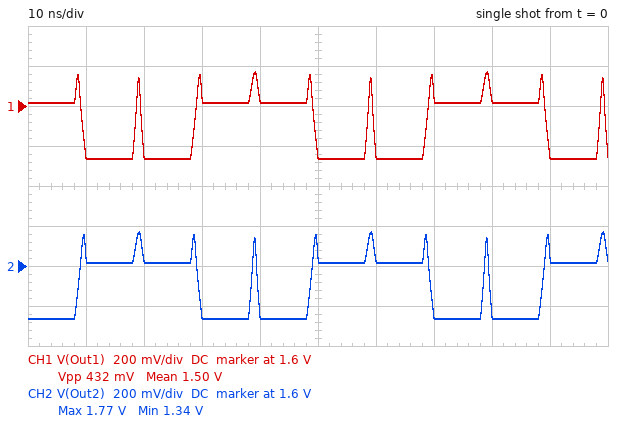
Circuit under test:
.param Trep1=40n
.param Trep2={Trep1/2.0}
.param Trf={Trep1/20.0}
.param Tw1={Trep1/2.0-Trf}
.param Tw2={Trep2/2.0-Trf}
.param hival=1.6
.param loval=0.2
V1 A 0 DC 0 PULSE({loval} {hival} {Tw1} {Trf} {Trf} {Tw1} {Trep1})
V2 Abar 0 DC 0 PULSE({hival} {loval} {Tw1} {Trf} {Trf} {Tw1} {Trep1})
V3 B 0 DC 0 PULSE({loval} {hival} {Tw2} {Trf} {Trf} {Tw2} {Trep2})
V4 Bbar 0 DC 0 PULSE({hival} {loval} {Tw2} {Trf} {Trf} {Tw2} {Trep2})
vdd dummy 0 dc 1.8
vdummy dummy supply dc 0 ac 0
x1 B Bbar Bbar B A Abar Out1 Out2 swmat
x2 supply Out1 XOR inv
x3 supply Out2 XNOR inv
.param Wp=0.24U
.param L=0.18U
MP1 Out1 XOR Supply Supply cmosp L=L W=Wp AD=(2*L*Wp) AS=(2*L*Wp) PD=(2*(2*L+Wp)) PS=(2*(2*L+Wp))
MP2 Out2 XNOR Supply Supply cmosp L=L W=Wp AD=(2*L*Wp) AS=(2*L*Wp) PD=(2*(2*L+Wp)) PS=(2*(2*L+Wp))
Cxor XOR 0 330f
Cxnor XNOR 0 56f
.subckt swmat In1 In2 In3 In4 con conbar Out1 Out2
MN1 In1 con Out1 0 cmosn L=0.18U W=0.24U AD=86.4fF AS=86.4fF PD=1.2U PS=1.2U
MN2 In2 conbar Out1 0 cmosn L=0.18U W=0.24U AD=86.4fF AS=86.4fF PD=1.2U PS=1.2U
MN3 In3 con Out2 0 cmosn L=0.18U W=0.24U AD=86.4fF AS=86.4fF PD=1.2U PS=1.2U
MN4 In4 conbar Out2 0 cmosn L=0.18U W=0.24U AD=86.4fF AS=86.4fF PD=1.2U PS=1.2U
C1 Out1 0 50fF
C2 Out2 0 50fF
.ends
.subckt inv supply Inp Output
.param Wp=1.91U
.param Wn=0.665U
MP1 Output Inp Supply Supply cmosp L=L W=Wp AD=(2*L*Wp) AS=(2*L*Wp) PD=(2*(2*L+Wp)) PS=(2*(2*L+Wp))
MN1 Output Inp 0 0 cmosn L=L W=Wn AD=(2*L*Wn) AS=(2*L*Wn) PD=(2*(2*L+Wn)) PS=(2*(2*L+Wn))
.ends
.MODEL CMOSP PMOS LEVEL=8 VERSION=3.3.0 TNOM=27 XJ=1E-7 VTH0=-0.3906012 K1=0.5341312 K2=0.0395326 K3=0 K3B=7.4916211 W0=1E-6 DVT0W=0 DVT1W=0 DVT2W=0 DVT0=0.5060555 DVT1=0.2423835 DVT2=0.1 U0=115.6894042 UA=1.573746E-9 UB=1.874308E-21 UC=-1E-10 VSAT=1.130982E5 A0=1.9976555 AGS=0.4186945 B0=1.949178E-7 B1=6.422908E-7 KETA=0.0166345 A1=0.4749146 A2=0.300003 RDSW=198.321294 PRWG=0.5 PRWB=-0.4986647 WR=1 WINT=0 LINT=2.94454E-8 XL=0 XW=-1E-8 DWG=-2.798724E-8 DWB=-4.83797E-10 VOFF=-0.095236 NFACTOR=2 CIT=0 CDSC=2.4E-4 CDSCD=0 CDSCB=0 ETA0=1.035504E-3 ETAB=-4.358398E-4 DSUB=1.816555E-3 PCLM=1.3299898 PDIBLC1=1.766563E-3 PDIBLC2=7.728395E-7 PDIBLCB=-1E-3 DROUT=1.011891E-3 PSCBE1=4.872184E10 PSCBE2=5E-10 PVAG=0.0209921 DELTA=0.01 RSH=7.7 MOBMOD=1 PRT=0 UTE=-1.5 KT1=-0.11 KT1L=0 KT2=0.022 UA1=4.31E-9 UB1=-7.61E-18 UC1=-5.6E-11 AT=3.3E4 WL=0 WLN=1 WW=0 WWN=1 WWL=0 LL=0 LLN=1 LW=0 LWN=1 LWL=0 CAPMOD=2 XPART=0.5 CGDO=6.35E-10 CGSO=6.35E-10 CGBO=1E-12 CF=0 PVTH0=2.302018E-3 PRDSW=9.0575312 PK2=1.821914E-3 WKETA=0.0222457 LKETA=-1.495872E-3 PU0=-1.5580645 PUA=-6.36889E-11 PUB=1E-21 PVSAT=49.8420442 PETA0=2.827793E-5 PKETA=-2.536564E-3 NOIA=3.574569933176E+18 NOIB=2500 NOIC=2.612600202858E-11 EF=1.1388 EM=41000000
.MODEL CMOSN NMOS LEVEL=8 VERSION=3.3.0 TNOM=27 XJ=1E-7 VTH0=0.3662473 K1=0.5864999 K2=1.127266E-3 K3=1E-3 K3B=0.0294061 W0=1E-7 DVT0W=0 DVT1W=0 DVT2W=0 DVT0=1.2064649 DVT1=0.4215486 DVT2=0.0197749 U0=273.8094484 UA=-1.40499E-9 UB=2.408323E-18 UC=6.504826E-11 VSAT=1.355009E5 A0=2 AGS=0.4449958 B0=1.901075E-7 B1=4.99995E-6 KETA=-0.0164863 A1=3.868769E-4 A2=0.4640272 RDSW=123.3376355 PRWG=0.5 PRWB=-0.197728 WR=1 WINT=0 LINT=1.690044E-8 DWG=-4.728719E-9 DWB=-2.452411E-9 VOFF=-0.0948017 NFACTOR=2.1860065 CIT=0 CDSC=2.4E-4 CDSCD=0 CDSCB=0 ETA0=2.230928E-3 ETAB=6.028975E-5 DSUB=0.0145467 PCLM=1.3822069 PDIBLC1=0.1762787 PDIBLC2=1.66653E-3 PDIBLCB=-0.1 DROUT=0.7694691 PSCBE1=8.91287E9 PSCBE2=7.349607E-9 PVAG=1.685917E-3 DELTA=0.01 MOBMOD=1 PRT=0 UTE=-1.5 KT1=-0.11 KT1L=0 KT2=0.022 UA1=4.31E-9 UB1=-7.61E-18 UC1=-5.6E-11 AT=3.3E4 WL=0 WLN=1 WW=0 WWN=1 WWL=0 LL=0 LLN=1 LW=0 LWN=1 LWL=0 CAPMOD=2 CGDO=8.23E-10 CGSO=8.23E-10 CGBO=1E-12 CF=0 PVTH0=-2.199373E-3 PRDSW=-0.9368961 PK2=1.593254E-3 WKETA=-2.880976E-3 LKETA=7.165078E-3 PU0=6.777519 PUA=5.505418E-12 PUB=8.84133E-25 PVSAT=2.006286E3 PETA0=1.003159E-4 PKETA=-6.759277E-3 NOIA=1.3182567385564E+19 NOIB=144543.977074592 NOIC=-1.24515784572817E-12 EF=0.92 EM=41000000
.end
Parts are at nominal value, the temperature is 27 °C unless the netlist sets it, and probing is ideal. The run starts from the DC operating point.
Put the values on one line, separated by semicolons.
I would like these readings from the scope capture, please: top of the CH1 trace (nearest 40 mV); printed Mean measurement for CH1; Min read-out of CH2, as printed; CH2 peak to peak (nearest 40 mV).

1.76 V; 1.50 V; 1.34 V; 440 mV
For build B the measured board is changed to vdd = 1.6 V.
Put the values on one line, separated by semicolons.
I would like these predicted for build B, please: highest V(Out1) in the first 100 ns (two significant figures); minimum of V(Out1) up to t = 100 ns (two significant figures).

1.6 V; 1.2 V
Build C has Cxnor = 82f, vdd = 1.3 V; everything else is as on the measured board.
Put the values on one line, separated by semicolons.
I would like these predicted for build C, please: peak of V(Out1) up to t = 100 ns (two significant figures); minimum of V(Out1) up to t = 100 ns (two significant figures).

1.3 V; 920 mV
